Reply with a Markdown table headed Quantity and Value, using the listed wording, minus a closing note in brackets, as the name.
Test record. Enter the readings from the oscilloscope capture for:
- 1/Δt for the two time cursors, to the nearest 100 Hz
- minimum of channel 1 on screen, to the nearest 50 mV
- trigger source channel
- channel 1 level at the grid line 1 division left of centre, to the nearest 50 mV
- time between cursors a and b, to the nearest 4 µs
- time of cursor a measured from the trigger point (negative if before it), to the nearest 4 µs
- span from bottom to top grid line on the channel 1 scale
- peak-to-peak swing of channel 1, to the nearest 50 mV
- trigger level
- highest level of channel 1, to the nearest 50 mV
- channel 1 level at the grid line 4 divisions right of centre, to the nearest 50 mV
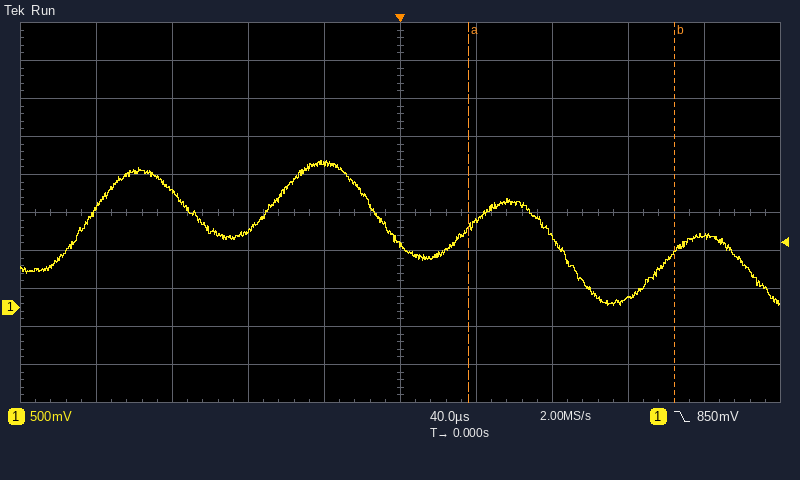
| Quantity | Value |
|---|---|
| 1/Δt for the two time cursors, to the nearest 100 Hz | 9.3 kHz |
| minimum of channel 1 on screen, to the nearest 50 mV | 50 mV |
| trigger source channel | channel 1 |
| channel 1 level at the grid line 1 division left of centre, to the nearest 50 mV | 1.90 V |
| time between cursors a and b, to the nearest 4 µs | 108 µs |
| time of cursor a measured from the trigger point (negative if before it), to the nearest 4 µs | +36 µs |
| span from bottom to top grid line on the channel 1 scale | 5 V |
| peak-to-peak swing of channel 1, to the nearest 50 mV | 1.90 V |
| trigger level | 850 mV |
| highest level of channel 1, to the nearest 50 mV | 1.95 V |
| channel 1 level at the grid line 4 divisions right of centre, to the nearest 50 mV | 950 mV |
